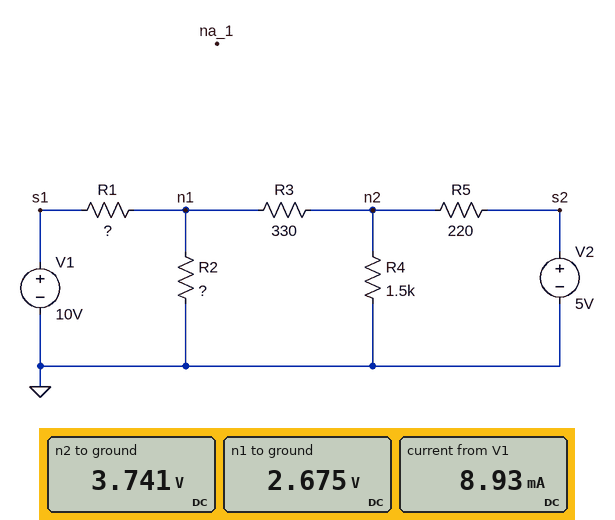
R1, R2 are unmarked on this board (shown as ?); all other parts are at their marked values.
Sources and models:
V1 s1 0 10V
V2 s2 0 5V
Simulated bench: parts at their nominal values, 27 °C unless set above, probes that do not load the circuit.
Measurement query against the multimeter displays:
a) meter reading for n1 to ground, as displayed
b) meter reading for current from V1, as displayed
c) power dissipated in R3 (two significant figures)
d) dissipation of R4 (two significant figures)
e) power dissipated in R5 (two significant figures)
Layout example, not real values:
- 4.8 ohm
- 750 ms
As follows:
- 2.675 V
- 8.93 mA
- 3.4 mW
- 9.3 mW
- 7.2 mW
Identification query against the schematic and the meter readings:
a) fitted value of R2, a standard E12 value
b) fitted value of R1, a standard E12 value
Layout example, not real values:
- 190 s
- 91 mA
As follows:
- 220 Ω
- 820 Ω
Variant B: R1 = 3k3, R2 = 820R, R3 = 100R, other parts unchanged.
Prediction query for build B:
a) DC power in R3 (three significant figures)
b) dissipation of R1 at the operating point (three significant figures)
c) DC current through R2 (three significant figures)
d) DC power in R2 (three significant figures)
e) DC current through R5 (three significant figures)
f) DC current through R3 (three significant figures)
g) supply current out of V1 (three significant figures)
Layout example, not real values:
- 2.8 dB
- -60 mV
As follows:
- 624 µW
- 12.3 mW
- 4.43 mA
- 16.1 mW
- 5.09 mA
- 2.50 mA
- 1.93 mA
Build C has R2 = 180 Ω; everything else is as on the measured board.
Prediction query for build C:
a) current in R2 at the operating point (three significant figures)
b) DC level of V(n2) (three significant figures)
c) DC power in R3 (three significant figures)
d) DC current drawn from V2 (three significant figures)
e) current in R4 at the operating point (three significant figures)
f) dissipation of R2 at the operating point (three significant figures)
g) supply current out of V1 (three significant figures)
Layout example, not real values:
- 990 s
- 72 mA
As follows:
- 13.1 mA
- 3.63 V
- 4.83 mW
- 6.24 mA
- 2.42 mA
- 31.1 mW
- 9.31 mA
